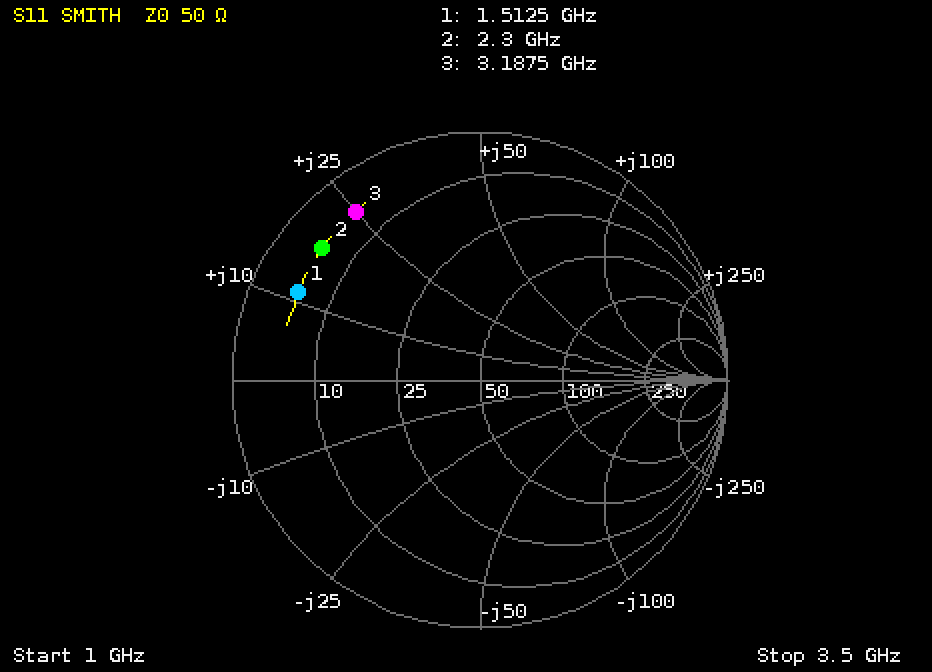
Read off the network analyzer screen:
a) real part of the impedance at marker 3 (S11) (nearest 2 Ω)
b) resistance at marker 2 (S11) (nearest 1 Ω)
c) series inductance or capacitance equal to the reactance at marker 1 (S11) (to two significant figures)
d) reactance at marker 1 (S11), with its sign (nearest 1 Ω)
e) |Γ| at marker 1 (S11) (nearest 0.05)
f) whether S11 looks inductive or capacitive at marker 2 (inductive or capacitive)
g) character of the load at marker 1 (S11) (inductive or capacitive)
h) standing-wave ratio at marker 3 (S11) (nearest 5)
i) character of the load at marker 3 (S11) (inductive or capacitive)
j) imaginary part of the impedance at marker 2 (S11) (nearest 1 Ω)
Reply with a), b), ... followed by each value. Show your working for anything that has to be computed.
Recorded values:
a) 6 Ω
b) 5 Ω
c) L = 11 Ω/(2π × 1.5125 GHz) ≈ 1.2 nH
d) +11 Ω
e) 0.80
f) inductive
g) inductive
h) 10
i) inductive
j) +18 Ω
